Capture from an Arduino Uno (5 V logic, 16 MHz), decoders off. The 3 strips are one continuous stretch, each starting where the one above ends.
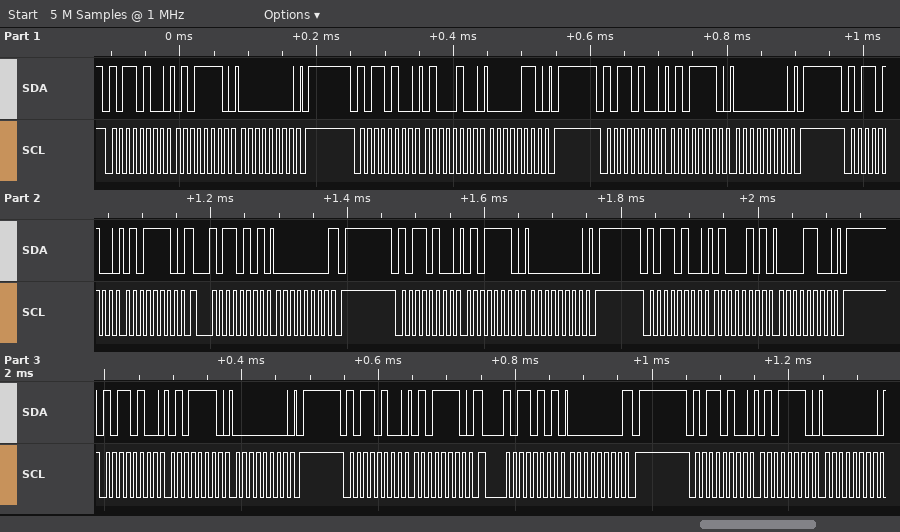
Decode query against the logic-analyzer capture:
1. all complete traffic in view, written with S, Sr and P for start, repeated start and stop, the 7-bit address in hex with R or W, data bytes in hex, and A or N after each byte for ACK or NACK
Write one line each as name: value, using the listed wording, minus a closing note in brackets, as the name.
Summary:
all complete traffic in view, written with S, Sr and P for start, repeated start and stop, the 7-bit address in hex with R or W, data bytes in hex, and A or N after each byte for ACK or NACK: S 5AW A 5E A 00 A P S 5AW A 44 A 06 A P S 5AW A 5E A 00 A P S 5AW A 5E A Sr 5AR A 00 N P S 5AW A 5E A 00 A P S 5AW A 45 A 0C A P S 5AW A 5E A 00 A P S 5AW A 5E A Sr 5AR A 00 N P S 5AW A 5E A 00 A
